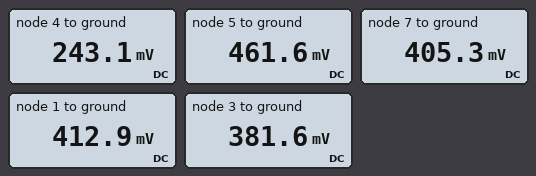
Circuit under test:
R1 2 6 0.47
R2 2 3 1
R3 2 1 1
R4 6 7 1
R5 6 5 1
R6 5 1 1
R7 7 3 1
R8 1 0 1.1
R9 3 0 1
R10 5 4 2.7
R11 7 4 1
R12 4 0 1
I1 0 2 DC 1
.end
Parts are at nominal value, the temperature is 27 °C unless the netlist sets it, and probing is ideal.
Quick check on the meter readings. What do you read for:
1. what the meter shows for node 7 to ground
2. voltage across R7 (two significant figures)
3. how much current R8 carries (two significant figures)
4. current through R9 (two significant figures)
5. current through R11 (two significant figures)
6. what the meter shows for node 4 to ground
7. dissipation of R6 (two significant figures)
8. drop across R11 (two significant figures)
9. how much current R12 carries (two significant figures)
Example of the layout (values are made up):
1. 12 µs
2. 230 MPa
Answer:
1. 405.3 mV
2. 24 mV
3. 380 mA
4. 380 mA
5. 160 mA
6. 243.1 mV
7. 2.4 mW
8. 160 mV
9. 240 mA
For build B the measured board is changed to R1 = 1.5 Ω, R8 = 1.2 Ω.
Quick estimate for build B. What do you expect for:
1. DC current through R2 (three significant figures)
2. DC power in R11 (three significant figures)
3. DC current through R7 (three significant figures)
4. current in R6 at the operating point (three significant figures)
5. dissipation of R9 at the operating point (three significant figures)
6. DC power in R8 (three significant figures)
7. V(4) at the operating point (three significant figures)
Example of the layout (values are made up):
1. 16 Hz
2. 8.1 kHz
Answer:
1. 420 mA
2. 22.9 mW
3. 19.5 mA
4. 4.92 mA
5. 160 mW
6. 165 mW
7. 229 mV
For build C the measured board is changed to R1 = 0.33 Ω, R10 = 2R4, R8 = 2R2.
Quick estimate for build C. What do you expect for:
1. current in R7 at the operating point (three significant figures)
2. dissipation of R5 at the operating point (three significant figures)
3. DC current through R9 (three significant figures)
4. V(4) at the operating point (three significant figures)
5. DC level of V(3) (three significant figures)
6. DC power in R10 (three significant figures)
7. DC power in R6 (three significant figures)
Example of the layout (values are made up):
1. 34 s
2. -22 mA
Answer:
1. 45.9 mA
2. 16.1 mW
3. 437 mA
4. 301 mV
5. 437 mV
6. 33.6 mW
7. 76.4 µW
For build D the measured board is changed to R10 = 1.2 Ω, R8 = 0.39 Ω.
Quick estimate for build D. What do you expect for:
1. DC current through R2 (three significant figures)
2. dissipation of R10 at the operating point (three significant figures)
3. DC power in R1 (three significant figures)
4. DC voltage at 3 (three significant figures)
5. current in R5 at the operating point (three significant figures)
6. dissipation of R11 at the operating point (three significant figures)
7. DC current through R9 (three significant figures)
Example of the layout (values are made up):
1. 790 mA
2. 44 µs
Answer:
1. 292 mA
2. 6.74 mW
3. 43.4 mW
4. 306 mV
5. 168 mA
6. 14.9 mW
7. 306 mA
